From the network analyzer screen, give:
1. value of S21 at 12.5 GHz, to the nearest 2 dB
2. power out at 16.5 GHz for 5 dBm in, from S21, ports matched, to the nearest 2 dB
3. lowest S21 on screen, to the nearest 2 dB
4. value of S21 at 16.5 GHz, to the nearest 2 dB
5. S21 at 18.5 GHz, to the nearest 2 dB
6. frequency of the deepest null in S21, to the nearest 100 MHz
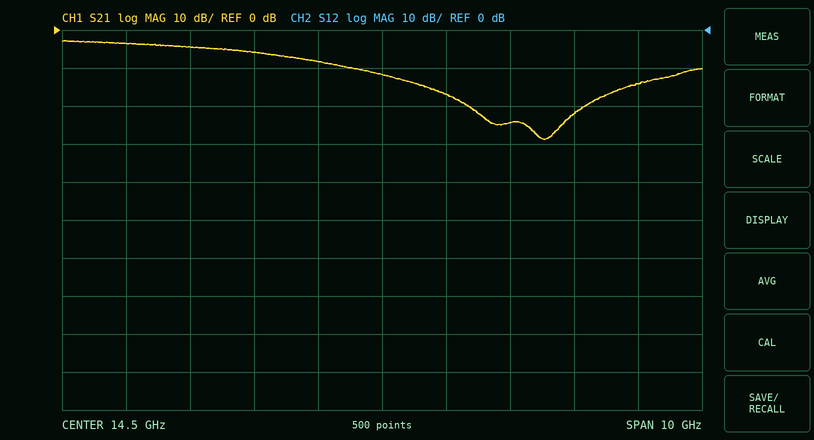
-6 dB
-20 dBm
-28 dB
-24 dB
-14 dB
17.0 GHz
